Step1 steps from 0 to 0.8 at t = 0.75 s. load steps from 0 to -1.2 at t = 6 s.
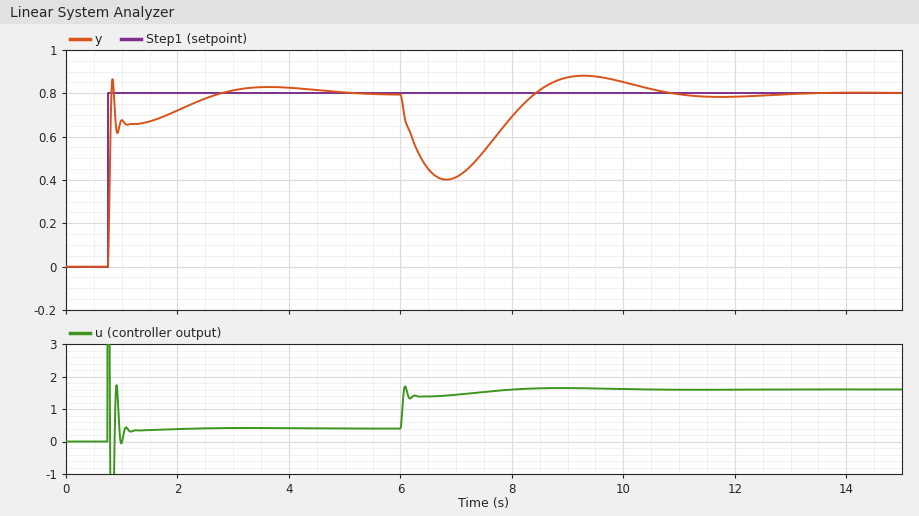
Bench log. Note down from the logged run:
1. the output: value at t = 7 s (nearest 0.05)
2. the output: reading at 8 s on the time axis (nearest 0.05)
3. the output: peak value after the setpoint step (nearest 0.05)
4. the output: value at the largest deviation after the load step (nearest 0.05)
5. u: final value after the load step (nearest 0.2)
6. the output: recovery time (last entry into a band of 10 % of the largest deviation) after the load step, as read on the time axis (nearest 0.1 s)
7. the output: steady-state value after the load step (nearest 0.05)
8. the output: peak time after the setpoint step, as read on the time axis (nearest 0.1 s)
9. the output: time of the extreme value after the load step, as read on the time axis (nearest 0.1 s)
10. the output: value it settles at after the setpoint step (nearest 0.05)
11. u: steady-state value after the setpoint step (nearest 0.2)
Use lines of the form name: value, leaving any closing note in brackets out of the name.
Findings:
the output: value at t = 7 s: 0.40
the output: reading at 8 s on the time axis: 0.70
the output: peak value after the setpoint step: 0.85
the output: value at the largest deviation after the load step: 0.40
u: final value after the load step: 1.6
the output: recovery time (last entry into a band of 10 % of the largest deviation) after the load step, as read on the time axis: 10.2 s
the output: steady-state value after the load step: 0.80
the output: peak time after the setpoint step, as read on the time axis: 0.8 s
the output: time of the extreme value after the load step, as read on the time axis: 6.8 s
the output: value it settles at after the setpoint step: 0.80
u: steady-state value after the setpoint step: 0.4
